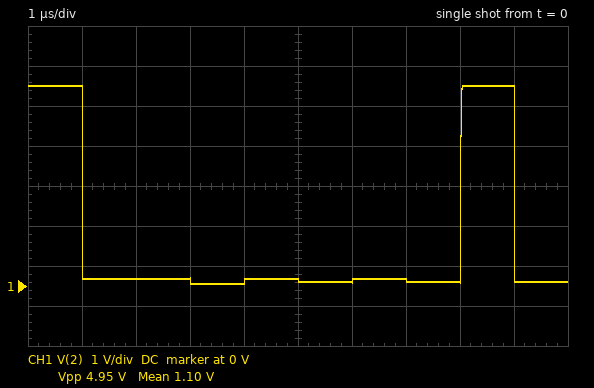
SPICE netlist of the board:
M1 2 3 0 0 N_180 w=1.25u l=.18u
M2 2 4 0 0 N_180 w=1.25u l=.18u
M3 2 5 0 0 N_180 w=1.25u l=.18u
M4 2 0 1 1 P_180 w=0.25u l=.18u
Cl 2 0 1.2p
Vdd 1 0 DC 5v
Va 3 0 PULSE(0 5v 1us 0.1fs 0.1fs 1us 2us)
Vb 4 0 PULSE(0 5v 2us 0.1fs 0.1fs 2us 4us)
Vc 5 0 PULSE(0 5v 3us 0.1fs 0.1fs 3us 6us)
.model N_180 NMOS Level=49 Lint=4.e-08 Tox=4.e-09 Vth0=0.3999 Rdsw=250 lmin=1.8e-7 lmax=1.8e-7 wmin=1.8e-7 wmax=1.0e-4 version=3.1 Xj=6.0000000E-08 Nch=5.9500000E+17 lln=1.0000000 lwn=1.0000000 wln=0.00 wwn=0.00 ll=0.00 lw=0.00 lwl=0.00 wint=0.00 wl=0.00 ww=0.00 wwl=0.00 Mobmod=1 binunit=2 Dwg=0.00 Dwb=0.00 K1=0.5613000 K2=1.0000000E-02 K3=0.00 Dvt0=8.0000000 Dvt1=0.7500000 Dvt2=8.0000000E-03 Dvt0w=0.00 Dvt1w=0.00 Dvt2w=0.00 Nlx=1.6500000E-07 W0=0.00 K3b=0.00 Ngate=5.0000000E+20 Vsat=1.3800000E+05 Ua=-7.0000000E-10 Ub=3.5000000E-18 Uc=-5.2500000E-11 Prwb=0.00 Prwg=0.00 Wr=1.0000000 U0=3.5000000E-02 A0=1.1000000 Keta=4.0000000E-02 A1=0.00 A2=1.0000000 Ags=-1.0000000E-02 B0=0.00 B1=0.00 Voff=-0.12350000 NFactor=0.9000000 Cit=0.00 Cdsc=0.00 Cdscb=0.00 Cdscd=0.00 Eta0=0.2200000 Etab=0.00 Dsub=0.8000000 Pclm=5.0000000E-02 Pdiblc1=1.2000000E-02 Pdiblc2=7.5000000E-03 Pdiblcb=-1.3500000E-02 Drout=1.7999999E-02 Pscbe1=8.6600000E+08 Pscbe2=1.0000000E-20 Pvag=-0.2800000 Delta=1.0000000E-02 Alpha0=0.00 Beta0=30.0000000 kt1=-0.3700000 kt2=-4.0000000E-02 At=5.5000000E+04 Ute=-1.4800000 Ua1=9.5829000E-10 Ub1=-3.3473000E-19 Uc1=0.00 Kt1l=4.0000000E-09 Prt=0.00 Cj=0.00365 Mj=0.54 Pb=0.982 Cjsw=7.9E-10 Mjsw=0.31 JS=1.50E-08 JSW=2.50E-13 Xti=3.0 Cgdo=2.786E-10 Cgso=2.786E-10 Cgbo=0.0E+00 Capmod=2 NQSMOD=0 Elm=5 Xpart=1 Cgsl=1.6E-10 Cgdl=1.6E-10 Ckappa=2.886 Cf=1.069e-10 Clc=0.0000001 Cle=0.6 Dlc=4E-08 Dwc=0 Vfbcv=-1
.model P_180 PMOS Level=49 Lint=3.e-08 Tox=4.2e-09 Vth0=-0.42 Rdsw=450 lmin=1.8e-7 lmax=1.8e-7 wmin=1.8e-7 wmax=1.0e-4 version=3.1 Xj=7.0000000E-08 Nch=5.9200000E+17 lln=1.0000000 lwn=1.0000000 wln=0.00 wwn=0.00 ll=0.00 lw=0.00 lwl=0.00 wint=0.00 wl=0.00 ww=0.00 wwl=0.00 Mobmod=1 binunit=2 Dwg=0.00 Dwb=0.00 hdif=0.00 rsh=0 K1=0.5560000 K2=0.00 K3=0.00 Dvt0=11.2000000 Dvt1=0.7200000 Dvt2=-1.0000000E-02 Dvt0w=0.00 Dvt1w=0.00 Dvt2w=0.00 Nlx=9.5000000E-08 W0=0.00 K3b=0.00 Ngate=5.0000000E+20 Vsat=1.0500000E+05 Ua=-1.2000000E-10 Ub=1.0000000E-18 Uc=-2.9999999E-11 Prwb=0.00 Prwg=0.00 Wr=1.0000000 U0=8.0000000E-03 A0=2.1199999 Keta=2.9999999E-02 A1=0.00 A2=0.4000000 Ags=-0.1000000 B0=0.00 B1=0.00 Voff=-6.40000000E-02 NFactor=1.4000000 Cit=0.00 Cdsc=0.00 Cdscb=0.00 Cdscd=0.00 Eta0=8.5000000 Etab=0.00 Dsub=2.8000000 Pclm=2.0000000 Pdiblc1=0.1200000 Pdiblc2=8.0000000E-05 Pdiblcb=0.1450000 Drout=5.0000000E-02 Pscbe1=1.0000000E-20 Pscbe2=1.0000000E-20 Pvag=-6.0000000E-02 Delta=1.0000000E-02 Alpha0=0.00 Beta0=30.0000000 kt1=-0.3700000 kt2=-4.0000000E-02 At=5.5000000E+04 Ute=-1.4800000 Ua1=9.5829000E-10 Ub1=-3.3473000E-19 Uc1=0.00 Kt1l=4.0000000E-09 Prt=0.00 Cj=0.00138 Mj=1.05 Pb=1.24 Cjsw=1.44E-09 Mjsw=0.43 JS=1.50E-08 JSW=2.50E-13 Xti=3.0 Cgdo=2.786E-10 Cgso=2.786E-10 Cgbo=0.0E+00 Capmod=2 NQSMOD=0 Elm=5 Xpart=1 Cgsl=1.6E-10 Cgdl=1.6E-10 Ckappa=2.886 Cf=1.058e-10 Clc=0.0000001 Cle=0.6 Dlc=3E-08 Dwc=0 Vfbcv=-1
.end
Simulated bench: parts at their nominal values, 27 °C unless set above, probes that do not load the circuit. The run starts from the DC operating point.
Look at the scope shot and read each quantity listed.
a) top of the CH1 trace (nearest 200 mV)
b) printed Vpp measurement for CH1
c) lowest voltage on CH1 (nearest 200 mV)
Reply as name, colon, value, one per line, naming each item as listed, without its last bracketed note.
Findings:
top of the CH1 trace: 5.0 V
printed Vpp measurement for CH1: 4.95 V
lowest voltage on CH1: 0 V
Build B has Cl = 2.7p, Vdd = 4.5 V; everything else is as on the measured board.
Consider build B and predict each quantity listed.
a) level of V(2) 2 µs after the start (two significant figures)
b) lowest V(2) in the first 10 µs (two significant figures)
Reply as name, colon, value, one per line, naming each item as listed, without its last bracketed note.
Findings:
level of V(2) 2 µs after the start: 160 mV
lowest V(2) in the first 10 µs: 49 mV
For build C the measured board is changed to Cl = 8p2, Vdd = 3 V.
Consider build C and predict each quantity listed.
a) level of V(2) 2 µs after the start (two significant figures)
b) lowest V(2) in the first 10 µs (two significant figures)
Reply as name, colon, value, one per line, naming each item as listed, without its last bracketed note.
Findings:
level of V(2) 2 µs after the start: 100 mV
lowest V(2) in the first 10 µs: 32 mV
